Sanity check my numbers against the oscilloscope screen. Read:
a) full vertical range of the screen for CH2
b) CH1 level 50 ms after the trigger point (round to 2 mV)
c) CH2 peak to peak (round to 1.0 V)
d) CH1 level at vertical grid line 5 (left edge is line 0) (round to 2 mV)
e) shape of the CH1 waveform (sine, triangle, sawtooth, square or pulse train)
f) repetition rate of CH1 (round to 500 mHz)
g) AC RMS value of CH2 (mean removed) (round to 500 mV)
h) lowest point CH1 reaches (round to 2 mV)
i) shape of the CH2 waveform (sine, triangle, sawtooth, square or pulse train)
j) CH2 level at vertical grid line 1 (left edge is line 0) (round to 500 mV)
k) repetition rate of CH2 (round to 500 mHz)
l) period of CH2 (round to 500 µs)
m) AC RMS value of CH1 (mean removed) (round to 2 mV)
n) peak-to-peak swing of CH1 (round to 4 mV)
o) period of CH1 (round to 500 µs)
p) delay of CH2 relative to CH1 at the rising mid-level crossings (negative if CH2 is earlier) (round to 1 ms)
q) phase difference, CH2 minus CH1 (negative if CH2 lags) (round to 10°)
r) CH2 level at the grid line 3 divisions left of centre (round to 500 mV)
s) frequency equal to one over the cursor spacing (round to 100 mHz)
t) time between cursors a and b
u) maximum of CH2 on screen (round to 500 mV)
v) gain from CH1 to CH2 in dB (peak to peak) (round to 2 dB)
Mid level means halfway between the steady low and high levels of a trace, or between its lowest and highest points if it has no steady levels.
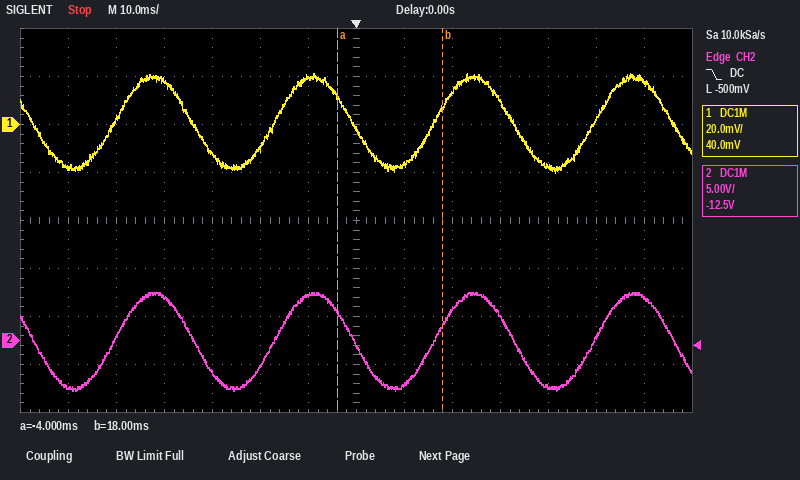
40 V
2 mV
10.0 V
-10 mV
sine
30.0 Hz
3.5 V
-20 mV
sine
-5.0 V
30.0 Hz
33.5 ms
14 mV
40 mV
33.5 ms
0 ms
0°
-3.5 V
45.5 Hz
22 ms
5.0 V
48 dB
